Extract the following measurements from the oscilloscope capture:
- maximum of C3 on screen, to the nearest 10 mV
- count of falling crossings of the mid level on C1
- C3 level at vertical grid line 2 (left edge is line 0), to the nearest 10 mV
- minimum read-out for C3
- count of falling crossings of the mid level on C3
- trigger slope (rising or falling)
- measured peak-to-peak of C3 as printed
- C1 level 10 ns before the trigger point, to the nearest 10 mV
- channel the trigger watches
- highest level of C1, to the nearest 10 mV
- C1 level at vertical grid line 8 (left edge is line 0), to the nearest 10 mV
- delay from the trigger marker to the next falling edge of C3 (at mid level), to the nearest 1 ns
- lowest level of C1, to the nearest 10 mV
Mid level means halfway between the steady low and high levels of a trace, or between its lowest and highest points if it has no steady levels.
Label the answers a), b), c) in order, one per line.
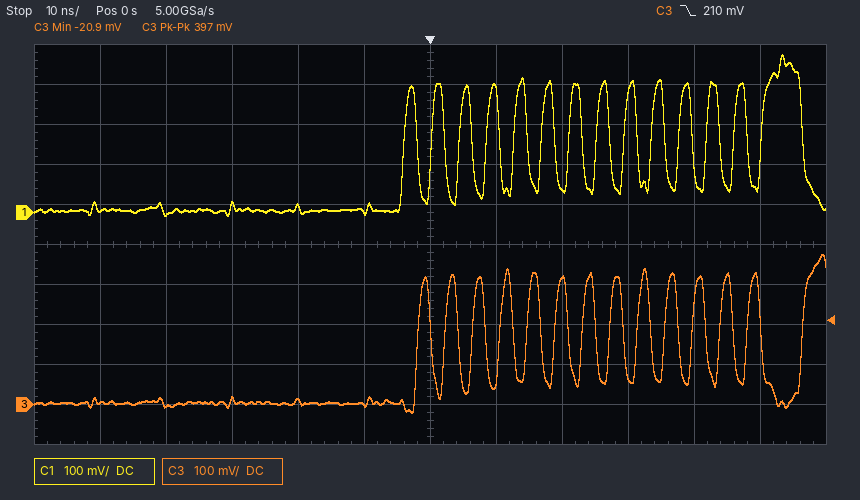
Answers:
a) 380 mV
b) 14
c) 0 mV
d) -20.9 mV
e) 13
f) falling
g) 397 mV
h) 0 mV
i) C3
j) 400 mV
k) 60 mV
l) 4 ns
m) -10 mV
